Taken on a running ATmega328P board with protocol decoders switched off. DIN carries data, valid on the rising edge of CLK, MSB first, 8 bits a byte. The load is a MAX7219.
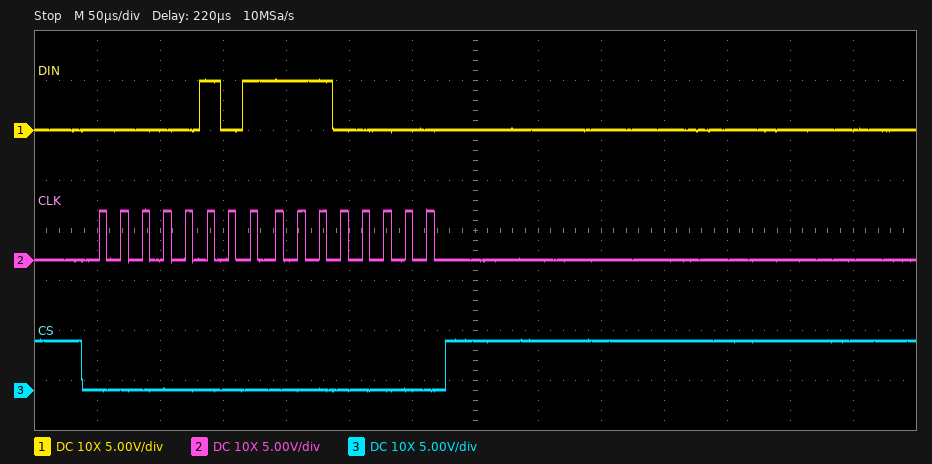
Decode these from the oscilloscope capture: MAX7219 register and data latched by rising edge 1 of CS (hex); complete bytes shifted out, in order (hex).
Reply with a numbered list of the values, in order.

1. register 0x5, data 0xE0
2. 05 E0
